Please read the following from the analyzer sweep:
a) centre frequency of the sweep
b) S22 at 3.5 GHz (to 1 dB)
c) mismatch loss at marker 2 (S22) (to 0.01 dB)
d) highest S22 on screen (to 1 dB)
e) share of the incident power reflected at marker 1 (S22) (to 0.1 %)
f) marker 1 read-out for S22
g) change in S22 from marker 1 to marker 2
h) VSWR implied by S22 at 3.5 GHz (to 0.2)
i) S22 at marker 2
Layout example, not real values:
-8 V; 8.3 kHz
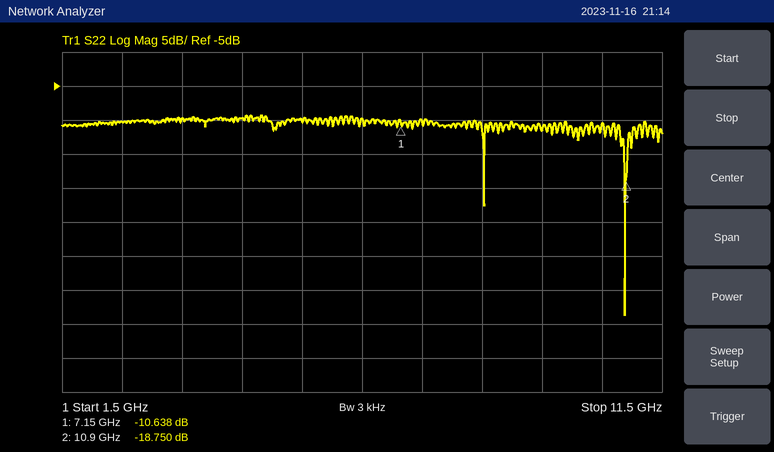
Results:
6.5 GHz; -10 dB; 0.06 dB; -9 dB; 8.6 %; -10.638 dB; -8.112 dB; 2.0; -18.750 dB
